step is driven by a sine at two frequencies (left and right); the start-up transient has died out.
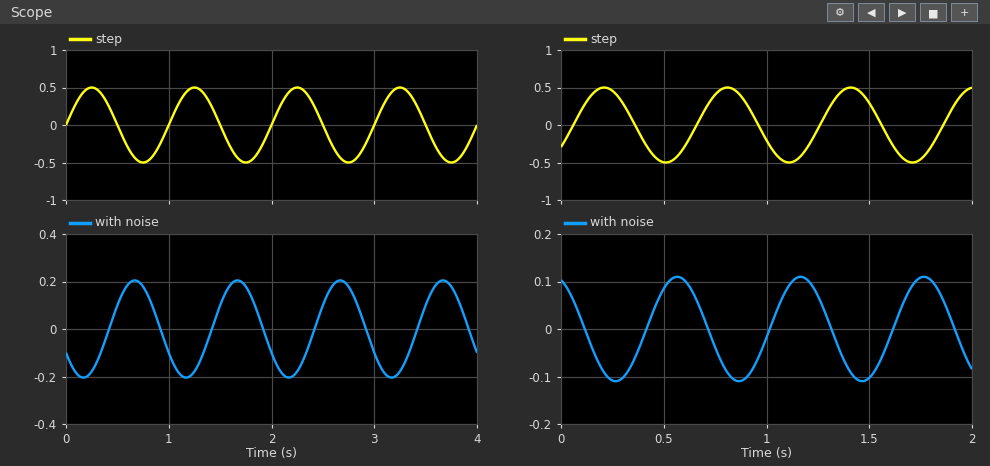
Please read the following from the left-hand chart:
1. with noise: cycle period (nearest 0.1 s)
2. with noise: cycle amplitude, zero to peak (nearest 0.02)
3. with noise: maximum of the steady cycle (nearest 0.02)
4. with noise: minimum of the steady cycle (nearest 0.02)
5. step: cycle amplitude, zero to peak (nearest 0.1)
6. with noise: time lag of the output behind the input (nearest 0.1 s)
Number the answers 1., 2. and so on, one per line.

1. 1.0 s
2. 0.20
3. 0.20
4. -0.20
5. 0.5
6. 0.4 s
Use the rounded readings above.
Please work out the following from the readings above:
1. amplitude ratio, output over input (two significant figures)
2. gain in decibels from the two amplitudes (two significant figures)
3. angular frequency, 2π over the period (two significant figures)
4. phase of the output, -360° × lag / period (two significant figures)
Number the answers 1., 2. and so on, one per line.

1. 0.40
2. -8.0 dB
3. 6.3 rad/s
4. -140°
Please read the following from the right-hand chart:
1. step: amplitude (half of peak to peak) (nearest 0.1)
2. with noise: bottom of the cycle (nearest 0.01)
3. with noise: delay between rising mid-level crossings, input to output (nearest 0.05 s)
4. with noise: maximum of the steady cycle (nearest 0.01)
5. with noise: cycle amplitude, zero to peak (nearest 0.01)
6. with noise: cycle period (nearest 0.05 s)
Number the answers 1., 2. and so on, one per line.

1. 0.5
2. -0.11
3. 0.35 s
4. 0.11
5. 0.11
6. 0.60 s
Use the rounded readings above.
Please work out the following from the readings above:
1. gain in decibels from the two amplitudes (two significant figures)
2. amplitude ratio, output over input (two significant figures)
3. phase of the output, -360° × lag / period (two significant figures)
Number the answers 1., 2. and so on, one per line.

1. -13 dB
2. 0.22
3. -210°
